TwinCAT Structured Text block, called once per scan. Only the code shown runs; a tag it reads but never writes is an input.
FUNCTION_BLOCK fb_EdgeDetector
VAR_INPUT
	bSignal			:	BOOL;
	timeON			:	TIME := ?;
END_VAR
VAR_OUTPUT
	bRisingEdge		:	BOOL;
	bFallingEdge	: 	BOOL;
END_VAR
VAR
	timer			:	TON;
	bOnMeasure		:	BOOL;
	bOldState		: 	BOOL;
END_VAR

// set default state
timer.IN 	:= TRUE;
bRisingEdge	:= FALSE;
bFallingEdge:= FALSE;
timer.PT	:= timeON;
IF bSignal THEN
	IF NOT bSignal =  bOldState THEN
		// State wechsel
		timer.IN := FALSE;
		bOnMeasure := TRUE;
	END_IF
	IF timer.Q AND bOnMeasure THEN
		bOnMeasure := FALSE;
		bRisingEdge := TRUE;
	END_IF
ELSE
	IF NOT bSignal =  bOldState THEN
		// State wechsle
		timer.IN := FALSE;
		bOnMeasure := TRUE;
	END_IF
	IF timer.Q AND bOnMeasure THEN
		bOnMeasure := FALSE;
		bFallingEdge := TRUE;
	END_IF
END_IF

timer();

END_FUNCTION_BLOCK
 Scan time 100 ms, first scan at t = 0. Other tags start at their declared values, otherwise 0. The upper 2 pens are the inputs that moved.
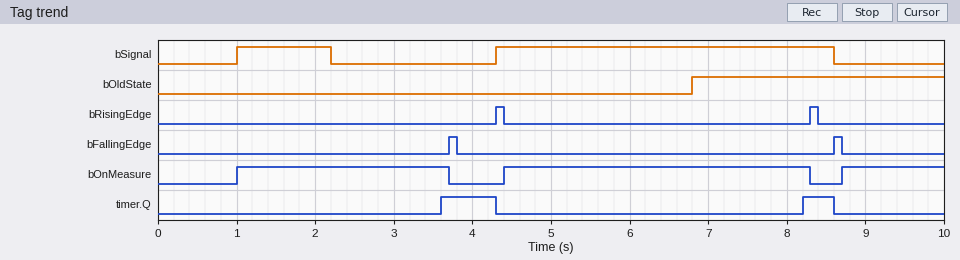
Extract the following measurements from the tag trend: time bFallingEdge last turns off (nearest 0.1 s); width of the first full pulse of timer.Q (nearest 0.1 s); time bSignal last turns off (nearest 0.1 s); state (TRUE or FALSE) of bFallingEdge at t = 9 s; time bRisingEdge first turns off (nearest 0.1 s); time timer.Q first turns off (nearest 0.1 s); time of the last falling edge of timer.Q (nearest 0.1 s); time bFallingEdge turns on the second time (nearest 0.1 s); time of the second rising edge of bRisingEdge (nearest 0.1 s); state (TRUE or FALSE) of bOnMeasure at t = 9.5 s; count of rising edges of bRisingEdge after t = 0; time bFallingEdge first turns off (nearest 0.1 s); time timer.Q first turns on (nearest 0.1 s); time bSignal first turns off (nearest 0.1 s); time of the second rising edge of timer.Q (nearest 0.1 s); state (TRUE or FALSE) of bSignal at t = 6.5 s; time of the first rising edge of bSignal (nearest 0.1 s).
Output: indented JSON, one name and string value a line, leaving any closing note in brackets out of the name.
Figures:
{
  "time bFallingEdge last turns off": "8.7 s",
  "width of the first full pulse of timer.Q": "0.7 s",
  "time bSignal last turns off": "8.6 s",
  "state (TRUE or FALSE) of bFallingEdge at t = 9 s": "FALSE",
  "time bRisingEdge first turns off": "4.4 s",
  "time timer.Q first turns off": "4.3 s",
  "time of the last falling edge of timer.Q": "8.6 s",
  "time bFallingEdge turns on the second time": "8.6 s",
  "time of the second rising edge of bRisingEdge": "8.3 s",
  "state (TRUE or FALSE) of bOnMeasure at t = 9.5 s": "TRUE",
  "count of rising edges of bRisingEdge after t = 0": "2",
  "time bFallingEdge first turns off": "3.8 s",
  "time timer.Q first turns on": "3.6 s",
  "time bSignal first turns off": "2.2 s",
  "time of the second rising edge of timer.Q": "8.2 s",
  "state (TRUE or FALSE) of bSignal at t = 6.5 s": "TRUE",
  "time of the first rising edge of bSignal": "1.0 s"
}
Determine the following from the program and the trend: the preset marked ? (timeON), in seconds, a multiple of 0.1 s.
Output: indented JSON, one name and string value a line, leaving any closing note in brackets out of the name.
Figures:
{
  "the preset marked ? (timeON), in seconds, a multiple of 0.1 s": "1.4 s"
}
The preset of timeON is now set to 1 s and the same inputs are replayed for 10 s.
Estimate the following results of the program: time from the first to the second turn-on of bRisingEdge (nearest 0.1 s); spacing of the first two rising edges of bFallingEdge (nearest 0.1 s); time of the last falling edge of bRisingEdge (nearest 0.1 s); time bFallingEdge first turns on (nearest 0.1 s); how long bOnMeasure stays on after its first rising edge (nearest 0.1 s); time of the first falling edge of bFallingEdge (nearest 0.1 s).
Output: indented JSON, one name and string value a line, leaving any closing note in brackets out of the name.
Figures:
{
  "time from the first to the second turn-on of bRisingEdge": "3.6 s",
  "spacing of the first two rising edges of bFallingEdge": "5.3 s",
  "time of the last falling edge of bRisingEdge": "8.0 s",
  "time bFallingEdge first turns on": "3.3 s",
  "how long bOnMeasure stays on after its first rising edge": "2.3 s",
  "time of the first falling edge of bFallingEdge": "3.4 s"
}
